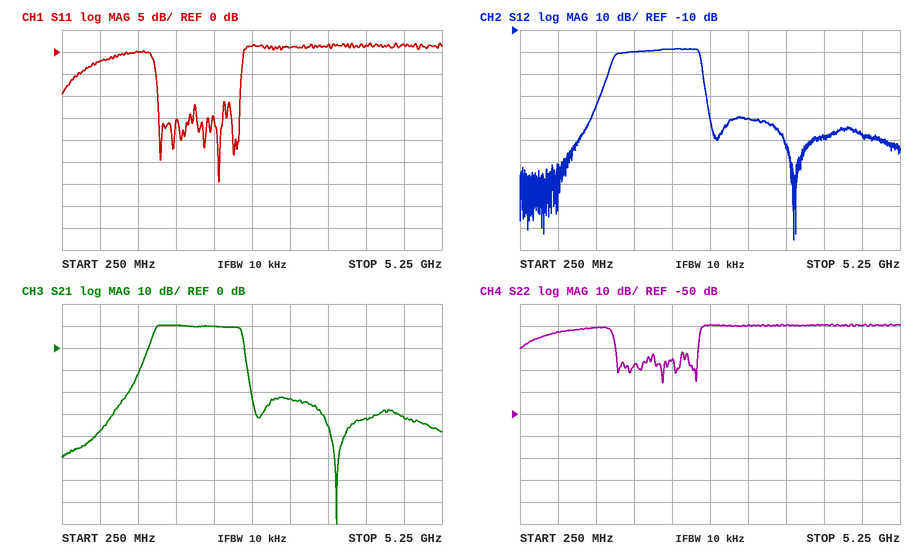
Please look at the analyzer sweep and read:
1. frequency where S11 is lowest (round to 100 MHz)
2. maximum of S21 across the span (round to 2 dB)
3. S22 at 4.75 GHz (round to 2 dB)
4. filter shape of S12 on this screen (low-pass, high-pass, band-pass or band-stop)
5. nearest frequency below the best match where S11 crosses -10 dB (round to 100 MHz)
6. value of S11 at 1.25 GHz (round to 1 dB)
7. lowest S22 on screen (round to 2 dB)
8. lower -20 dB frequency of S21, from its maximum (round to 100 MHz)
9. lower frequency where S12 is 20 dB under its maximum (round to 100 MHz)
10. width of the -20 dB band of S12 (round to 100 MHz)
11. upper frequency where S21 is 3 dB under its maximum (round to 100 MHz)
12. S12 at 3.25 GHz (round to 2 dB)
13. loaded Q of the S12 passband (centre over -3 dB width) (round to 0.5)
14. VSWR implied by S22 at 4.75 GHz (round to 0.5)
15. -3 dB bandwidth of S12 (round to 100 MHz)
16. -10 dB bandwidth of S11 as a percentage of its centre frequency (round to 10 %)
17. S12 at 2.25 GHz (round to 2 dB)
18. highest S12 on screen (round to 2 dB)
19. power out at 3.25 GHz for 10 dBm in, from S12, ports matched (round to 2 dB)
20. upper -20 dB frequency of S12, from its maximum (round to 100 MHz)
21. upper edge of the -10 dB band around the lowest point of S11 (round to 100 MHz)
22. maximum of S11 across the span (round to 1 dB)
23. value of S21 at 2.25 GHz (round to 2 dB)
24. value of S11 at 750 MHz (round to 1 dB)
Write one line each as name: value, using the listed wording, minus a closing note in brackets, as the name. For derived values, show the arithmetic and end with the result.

frequency where S11 is lowest: 2.3 GHz
maximum of S21 across the span: 10 dB
S22 at 4.75 GHz: -10 dB
filter shape of S12 on this screen: band-pass
nearest frequency below the best match where S11 crosses -10 dB: 1.5 GHz
value of S11 at 1.25 GHz: 0 dB
lowest S22 on screen: -36 dB
lower -20 dB frequency of S21, from its maximum: 1.3 GHz
lower frequency where S12 is 20 dB under its maximum: 1.3 GHz
width of the -20 dB band of S12: 2.7 GHz − 1.3 GHz = 1.4 GHz
upper frequency where S21 is 3 dB under its maximum: 2.6 GHz
S12 at 3.25 GHz: -50 dB
loaded Q of the S12 passband (centre over -3 dB width): 2.05 GHz / 1.1 GHz ≈ 1.86, so 2.0 to the nearest 0.5
VSWR implied by S22 at 4.75 GHz: |Γ| = 10^(-10/20) = 0.3162; VSWR = (1 + 0.3162)/(1 − 0.3162) ≈ 1.92, so 2.0 to the nearest 0.5
-3 dB bandwidth of S12: 2.6 GHz − 1.5 GHz = 1.1 GHz
-10 dB bandwidth of S11 as a percentage of its centre frequency: 1.1 GHz / 2.05 GHz ≈ 53.7 %, so 50 % to the nearest 10 %
S12 at 2.25 GHz: -18 dB
highest S12 on screen: -18 dB
power out at 3.25 GHz for 10 dBm in, from S12, ports matched: 10 dBm + (-50 dB) = -40 dBm
upper -20 dB frequency of S12, from its maximum: 2.7 GHz
upper edge of the -10 dB band around the lowest point of S11: 2.6 GHz
maximum of S11 across the span: 2 dB
value of S21 at 2.25 GHz: 10 dB
value of S11 at 750 MHz: -2 dB
